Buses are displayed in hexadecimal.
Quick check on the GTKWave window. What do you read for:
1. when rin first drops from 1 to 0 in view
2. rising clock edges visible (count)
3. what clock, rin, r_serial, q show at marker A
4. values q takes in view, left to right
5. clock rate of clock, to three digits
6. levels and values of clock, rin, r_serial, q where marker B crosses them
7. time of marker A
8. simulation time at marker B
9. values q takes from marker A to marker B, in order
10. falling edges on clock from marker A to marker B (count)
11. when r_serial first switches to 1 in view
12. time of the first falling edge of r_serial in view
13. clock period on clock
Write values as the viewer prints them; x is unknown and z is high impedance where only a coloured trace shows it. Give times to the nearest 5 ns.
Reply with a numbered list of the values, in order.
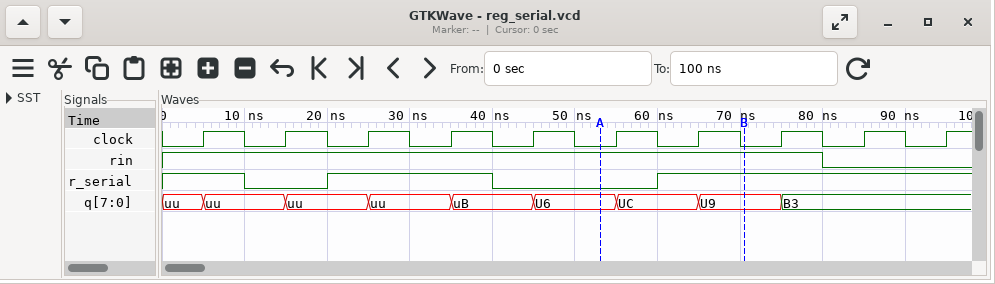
1. 80 ns
2. 10
3. clock=0, rin=1, r_serial=0, q=U6
4. uu, uu, uu, uu, uB, U6, UC, U9, B3
5. 100 MHz
6. clock=0, rin=1, r_serial=1, q=U9
7. 55 ns
8. 70 ns
9. U6, UC, U9
10. 2
11. 20 ns
12. 10 ns
13. 10 ns
